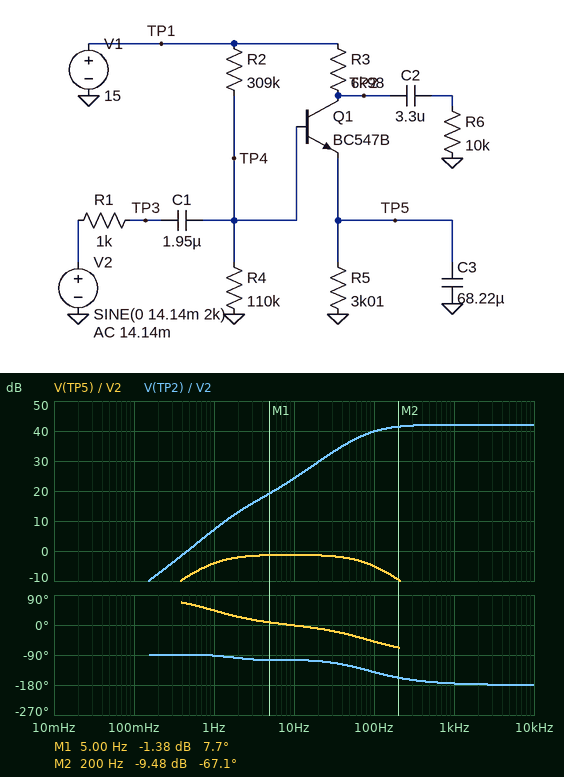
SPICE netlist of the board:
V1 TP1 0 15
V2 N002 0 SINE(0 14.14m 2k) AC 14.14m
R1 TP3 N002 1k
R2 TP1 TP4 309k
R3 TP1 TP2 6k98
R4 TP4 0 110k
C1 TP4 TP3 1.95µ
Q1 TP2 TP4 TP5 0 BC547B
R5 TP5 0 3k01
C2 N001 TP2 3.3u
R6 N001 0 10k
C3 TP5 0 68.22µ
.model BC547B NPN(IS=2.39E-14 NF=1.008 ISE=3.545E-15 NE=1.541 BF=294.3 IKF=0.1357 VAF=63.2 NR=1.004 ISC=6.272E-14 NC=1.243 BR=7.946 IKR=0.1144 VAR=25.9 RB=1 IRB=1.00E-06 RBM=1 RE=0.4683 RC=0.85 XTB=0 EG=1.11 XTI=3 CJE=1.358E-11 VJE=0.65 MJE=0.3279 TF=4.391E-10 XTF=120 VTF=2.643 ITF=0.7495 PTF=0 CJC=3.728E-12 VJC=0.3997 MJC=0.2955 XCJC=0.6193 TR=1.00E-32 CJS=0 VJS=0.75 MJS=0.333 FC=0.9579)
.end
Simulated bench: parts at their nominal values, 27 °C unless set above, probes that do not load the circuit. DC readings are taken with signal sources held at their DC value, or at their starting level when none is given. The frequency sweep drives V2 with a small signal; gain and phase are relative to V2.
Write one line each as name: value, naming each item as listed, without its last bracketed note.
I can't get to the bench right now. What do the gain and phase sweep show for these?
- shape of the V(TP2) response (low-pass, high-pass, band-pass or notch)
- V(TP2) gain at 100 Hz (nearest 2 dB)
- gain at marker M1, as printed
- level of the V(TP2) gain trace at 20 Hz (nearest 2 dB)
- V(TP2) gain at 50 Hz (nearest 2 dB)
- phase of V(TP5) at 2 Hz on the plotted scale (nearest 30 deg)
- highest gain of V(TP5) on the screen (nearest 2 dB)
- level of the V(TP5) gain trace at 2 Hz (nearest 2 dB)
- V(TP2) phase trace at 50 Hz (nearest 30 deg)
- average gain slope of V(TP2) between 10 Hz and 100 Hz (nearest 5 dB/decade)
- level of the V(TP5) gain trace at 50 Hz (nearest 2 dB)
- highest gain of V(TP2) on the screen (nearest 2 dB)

shape of the V(TP2) response: high-pass
V(TP2) gain at 100 Hz: 40 dB
gain at marker M1, as printed: -1.38 dB
level of the V(TP2) gain trace at 20 Hz: 30 dB
V(TP2) gain at 50 Hz: 36 dB
phase of V(TP5) at 2 Hz on the plotted scale: 30 deg
highest gain of V(TP5) on the screen: -2 dB
level of the V(TP5) gain trace at 2 Hz: -2 dB
V(TP2) phase trace at 50 Hz: -120 deg
average gain slope of V(TP2) between 10 Hz and 100 Hz: 15 dB/decade
level of the V(TP5) gain trace at 50 Hz: -2 dB
highest gain of V(TP2) on the screen: 42 dB
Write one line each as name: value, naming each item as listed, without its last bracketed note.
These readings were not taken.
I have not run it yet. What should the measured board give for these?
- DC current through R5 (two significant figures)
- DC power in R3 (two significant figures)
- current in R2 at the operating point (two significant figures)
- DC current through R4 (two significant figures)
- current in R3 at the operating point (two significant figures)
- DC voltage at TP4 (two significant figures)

DC current through R5: 1.0 mA
DC power in R3: 7.0 mW
current in R2 at the operating point: 37 µA
DC current through R4: 33 µA
current in R3 at the operating point: 1.0 mA
DC voltage at TP4: 3.7 V
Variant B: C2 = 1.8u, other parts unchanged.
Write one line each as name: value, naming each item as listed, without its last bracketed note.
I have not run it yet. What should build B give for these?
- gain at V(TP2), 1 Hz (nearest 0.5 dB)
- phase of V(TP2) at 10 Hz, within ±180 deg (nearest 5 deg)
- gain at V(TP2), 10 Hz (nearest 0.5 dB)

gain at V(TP2), 1 Hz: 7.5 dB
phase of V(TP2) at 10 Hz, within ±180 deg: -110 deg
gain at V(TP2), 10 Hz: 25.0 dB
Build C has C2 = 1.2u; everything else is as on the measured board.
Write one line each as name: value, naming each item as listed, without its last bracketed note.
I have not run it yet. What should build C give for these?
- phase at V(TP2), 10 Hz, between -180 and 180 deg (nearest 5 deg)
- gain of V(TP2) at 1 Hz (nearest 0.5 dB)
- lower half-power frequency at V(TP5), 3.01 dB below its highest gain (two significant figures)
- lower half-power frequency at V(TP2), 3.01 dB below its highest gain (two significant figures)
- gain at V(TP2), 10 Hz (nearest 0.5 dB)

phase at V(TP2), 10 Hz, between -180 and 180 deg: -110 deg
gain of V(TP2) at 1 Hz: 7.5 dB
lower half-power frequency at V(TP5), 3.01 dB below its highest gain: 950 mHz
lower half-power frequency at V(TP2), 3.01 dB below its highest gain: 82 Hz
gain at V(TP2), 10 Hz: 26.0 dB
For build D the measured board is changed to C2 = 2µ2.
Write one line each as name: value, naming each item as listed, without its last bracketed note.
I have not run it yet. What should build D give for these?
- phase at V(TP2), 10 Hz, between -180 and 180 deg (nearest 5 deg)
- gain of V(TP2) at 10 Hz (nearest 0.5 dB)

phase at V(TP2), 10 Hz, between -180 and 180 deg: -110 deg
gain of V(TP2) at 10 Hz: 24.5 dB
